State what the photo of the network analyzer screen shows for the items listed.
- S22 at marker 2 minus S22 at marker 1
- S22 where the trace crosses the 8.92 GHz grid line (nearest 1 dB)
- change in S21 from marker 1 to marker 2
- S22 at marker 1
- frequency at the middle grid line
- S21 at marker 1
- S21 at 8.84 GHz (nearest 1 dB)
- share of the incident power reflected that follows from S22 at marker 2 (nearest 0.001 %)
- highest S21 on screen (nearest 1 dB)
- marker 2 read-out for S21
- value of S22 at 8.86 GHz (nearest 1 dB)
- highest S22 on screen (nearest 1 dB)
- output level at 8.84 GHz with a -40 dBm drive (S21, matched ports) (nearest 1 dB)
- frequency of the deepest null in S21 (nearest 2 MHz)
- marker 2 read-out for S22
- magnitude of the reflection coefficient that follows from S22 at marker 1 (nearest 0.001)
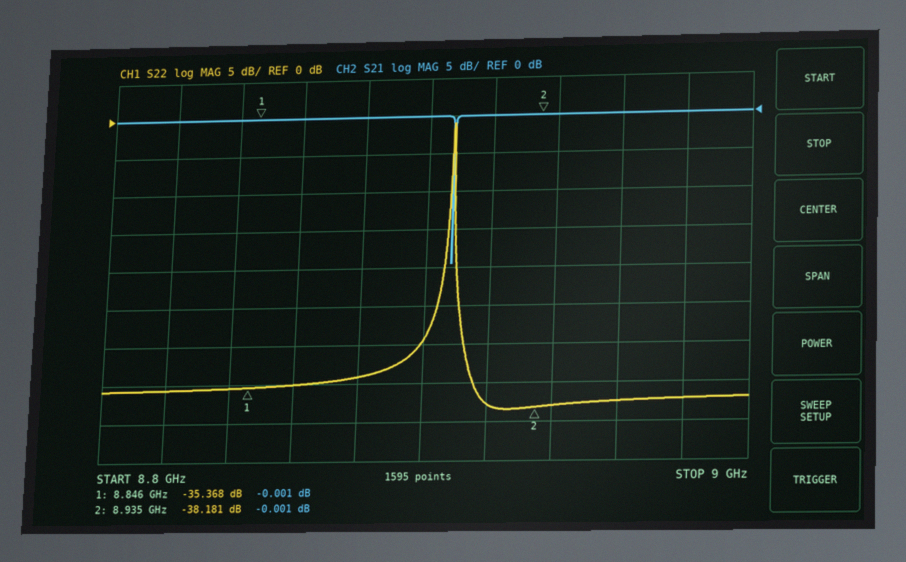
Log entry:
-2.813 dB
-38 dB
0.000 dB
-35.368 dB
8.9 GHz
-0.001 dB
0 dB
0.015 %
0 dB
-0.001 dB
-35 dB
-1 dB
-40 dBm
8.908 GHz
-38.181 dB
0.017
